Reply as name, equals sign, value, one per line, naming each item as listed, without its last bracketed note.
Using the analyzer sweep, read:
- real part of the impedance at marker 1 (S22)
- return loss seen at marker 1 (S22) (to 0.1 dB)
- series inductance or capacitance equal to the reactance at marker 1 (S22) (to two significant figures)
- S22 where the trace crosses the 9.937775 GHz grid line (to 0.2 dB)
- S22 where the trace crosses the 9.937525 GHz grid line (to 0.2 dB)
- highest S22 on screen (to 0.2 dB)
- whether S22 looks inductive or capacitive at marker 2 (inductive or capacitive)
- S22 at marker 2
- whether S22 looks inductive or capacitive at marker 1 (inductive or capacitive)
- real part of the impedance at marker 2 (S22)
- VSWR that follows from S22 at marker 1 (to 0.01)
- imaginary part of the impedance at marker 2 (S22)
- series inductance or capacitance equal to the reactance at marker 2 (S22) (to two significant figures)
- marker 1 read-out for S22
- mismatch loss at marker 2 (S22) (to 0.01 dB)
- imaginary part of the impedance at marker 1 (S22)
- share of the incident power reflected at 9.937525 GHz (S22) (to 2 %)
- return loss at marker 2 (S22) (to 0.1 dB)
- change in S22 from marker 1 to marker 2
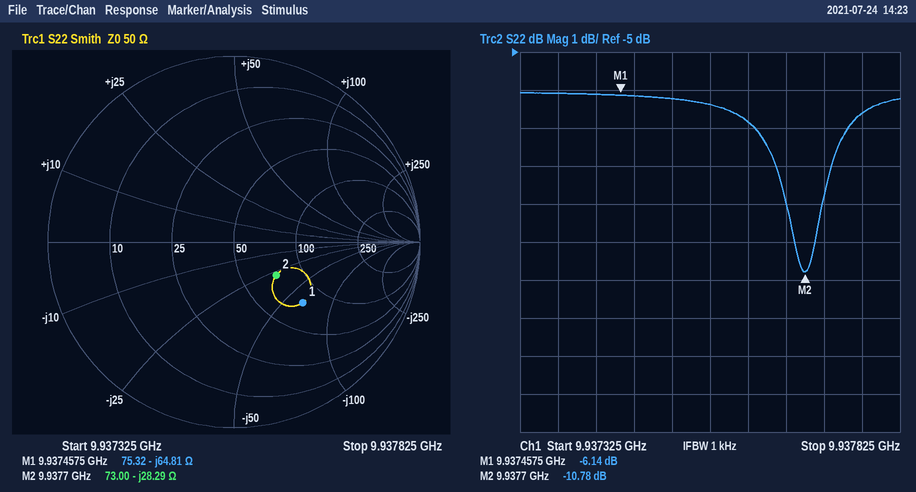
real part of the impedance at marker 1 = 75.32 Ω
return loss seen at marker 1 (S22) = 6.1 dB
series inductance or capacitance equal to the reactance at marker 1 (S22) = 250 fF
S22 where the trace crosses the 9.937775 GHz grid line = -6.6 dB
S22 where the trace crosses the 9.937525 GHz grid line = -6.2 dB
highest S22 on screen = -6.0 dB
whether S22 looks inductive or capacitive at marker 2 = capacitive
S22 at marker 2 = -10.78 dB
whether S22 looks inductive or capacitive at marker 1 = capacitive
real part of the impedance at marker 2 = 73.00 Ω
VSWR that follows from S22 at marker 1 = 2.95
imaginary part of the impedance at marker 2 = -28.29 Ω
series inductance or capacitance equal to the reactance at marker 2 (S22) = 570 fF
marker 1 read-out for S22 = -6.14 dB
mismatch loss at marker 2 (S22) = 0.38 dB
imaginary part of the impedance at marker 1 = -64.81 Ω
share of the incident power reflected at 9.937525 GHz (S22) = 24 %
return loss at marker 2 (S22) = 10.8 dB
change in S22 from marker 1 to marker 2 = -4.64 dB
